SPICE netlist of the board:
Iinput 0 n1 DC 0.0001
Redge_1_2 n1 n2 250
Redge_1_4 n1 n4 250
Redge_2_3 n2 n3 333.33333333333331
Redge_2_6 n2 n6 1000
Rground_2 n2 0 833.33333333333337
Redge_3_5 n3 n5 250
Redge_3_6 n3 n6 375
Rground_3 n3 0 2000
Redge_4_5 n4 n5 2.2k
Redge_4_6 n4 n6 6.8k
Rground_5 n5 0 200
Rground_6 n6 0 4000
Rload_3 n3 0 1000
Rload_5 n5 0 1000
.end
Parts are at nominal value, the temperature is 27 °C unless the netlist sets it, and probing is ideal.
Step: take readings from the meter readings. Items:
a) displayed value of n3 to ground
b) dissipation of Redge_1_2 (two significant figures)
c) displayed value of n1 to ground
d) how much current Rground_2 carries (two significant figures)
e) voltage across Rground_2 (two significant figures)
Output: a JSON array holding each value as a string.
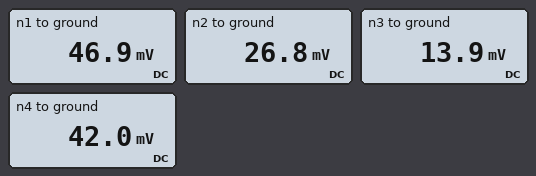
["13.9 mV", "1.6 µW", "46.9 mV", "32 µA", "27 mV"]
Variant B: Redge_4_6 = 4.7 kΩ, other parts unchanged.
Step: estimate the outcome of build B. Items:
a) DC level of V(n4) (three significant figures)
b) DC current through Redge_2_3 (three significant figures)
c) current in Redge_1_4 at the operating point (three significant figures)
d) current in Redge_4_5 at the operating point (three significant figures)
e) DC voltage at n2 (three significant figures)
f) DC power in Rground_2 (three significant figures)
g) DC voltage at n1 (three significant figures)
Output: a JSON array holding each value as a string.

["41.4 mV", "38.3 µA", "20.6 µA", "15.6 µA", "26.7 mV", "854 nW", "46.5 mV"]
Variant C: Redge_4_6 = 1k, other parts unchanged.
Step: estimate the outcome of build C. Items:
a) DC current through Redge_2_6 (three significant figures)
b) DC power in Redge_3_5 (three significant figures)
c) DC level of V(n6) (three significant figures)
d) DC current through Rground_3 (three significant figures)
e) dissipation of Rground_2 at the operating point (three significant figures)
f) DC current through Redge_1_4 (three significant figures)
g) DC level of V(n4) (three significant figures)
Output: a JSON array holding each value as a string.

["5.42 µA", "212 nW", "20.4 mV", "7.17 µA", "801 nW", "29.1 µA", "36.3 mV"]
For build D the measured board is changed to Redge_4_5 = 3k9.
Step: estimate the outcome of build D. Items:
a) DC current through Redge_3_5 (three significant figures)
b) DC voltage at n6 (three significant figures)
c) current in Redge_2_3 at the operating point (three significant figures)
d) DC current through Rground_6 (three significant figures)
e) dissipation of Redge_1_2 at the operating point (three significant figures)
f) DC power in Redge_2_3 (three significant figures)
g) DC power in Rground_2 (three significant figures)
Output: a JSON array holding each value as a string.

["30.2 µA", "18.0 mV", "41.7 µA", "4.49 µA", "1.84 µW", "581 nW", "953 nW"]
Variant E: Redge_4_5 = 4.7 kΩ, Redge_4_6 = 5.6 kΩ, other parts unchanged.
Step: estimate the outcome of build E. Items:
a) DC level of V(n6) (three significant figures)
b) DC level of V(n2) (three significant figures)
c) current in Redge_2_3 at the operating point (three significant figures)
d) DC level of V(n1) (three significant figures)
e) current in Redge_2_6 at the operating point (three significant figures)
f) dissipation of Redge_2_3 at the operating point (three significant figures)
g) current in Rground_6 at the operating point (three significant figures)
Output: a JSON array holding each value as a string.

["18.4 mV", "28.5 mV", "42.2 µA", "50.1 mV", "10.1 µA", "593 nW", "4.59 µA"]
